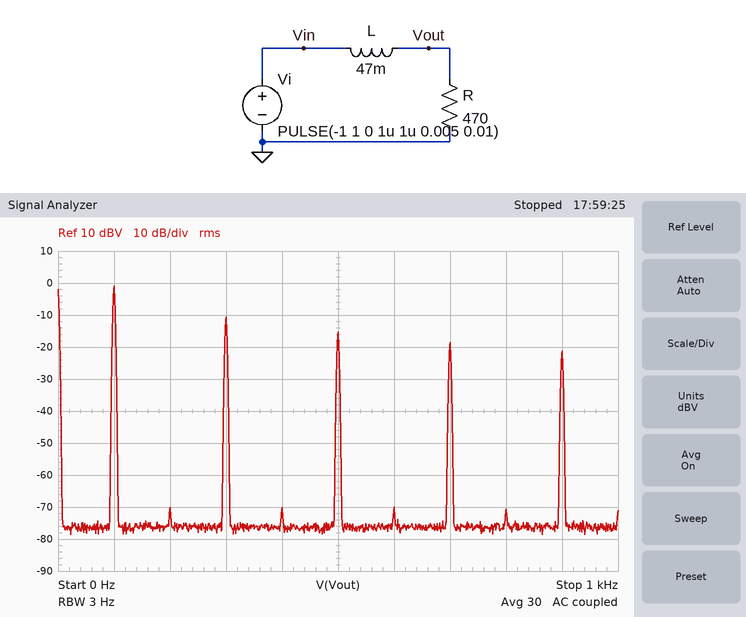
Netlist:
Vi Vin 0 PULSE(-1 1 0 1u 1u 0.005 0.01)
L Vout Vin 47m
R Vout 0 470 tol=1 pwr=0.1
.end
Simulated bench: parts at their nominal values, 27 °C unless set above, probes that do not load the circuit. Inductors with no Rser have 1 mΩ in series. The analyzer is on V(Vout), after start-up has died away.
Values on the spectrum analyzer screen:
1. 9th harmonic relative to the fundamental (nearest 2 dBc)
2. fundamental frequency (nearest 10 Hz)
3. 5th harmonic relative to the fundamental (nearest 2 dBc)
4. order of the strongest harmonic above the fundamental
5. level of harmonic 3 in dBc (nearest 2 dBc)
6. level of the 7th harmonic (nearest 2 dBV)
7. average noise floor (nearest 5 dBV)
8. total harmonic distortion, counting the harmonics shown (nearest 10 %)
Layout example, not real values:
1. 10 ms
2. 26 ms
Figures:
1. -20 dBc
2. 100 Hz
3. -14 dBc
4. 3
5. -10 dBc
6. -18 dBV
7. -75 dBV
8. 40 %
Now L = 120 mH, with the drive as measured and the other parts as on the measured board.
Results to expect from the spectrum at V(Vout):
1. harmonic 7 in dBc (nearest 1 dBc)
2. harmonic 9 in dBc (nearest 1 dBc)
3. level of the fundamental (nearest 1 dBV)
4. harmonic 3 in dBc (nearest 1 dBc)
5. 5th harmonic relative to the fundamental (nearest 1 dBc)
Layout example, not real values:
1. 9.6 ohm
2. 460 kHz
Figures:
1. -20 dBc
2. -24 dBc
3. -1 dBV
4. -10 dBc
5. -16 dBc
